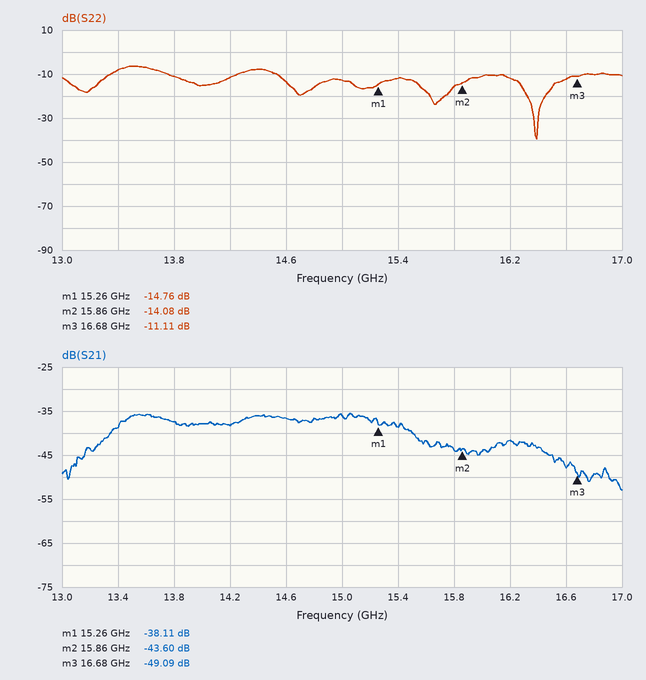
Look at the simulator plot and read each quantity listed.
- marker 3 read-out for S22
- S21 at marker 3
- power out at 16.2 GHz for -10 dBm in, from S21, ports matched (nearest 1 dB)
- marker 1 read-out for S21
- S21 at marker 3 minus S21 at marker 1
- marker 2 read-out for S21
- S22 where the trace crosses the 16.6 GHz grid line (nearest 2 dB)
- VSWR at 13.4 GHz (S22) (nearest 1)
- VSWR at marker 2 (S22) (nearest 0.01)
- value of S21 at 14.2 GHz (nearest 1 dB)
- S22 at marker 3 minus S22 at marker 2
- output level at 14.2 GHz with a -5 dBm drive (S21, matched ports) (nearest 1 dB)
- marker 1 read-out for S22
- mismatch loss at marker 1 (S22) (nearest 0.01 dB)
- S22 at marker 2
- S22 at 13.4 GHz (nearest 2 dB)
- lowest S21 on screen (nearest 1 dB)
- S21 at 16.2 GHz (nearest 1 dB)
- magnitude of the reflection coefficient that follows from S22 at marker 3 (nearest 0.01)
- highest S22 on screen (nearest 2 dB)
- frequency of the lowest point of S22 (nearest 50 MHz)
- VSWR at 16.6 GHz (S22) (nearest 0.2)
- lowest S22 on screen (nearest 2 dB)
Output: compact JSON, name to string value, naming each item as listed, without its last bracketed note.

{"marker 3 read-out for S22": "-11.11 dB", "S21 at marker 3": "-49.09 dB", "power out at 16.2 GHz for -10 dBm in, from S21, ports matched": "-52 dBm", "marker 1 read-out for S21": "-38.11 dB", "S21 at marker 3 minus S21 at marker 1": "-10.98 dB", "marker 2 read-out for S21": "-43.60 dB", "S22 where the trace crosses the 16.6 GHz grid line": "-12 dB", "VSWR at 13.4 GHz (S22)": "2", "VSWR at marker 2 (S22)": "1.49", "value of S21 at 14.2 GHz": "-38 dB", "S22 at marker 3 minus S22 at marker 2": "2.97 dB", "output level at 14.2 GHz with a -5 dBm drive (S21, matched ports)": "-43 dBm", "marker 1 read-out for S22": "-14.76 dB", "mismatch loss at marker 1 (S22)": "0.15 dB", "S22 at marker 2": "-14.08 dB", "S22 at 13.4 GHz": "-8 dB", "lowest S21 on screen": "-53 dB", "S21 at 16.2 GHz": "-42 dB", "magnitude of the reflection coefficient that follows from S22 at marker 3": "0.28", "highest S22 on screen": "-6 dB", "frequency of the lowest point of S22": "16.40 GHz", "VSWR at 16.6 GHz (S22)": "1.6", "lowest S22 on screen": "-40 dB"}
